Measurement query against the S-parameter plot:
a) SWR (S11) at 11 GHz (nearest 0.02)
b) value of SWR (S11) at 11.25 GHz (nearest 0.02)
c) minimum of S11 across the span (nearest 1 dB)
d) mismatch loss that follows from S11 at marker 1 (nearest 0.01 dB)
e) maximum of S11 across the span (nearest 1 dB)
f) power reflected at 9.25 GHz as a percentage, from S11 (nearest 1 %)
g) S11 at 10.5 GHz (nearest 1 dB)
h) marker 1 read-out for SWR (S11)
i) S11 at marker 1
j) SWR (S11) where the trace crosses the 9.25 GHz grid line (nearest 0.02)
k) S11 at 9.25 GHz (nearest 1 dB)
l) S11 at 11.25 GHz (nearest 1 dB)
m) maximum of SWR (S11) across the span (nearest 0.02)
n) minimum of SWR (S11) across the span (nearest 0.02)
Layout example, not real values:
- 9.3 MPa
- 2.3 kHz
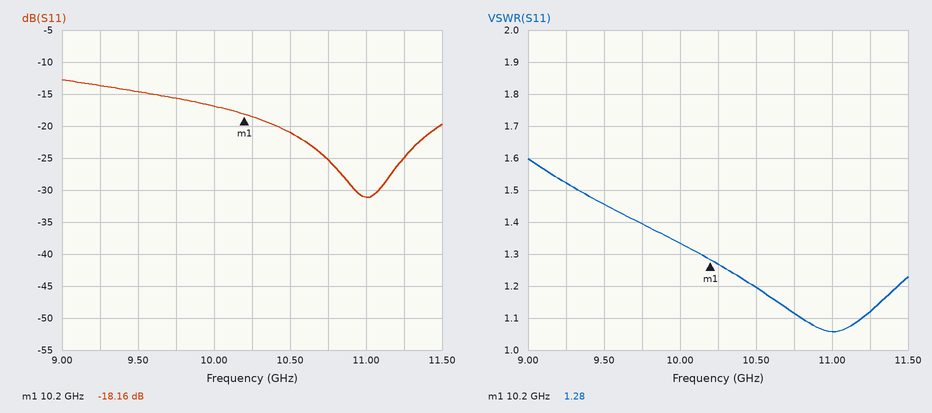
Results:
- 1.06
- 1.12
- -31 dB
- 0.07 dB
- -13 dB
- 4 %
- -21 dB
- 1.28
- -18.16 dB
- 1.52
- -14 dB
- -25 dB
- 1.60
- 1.06
